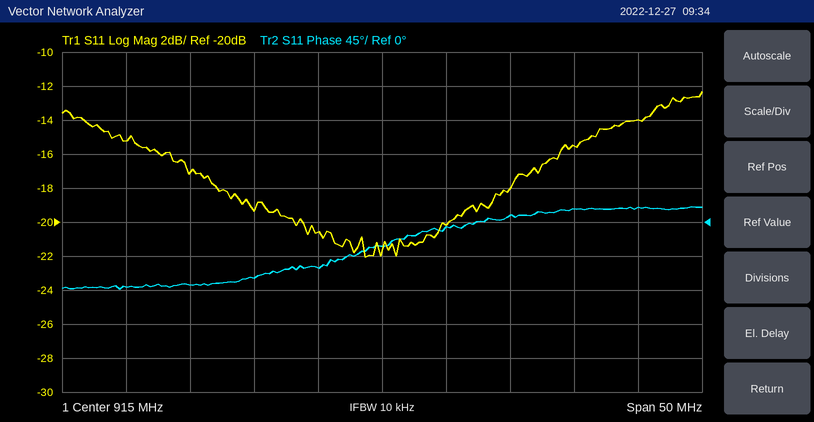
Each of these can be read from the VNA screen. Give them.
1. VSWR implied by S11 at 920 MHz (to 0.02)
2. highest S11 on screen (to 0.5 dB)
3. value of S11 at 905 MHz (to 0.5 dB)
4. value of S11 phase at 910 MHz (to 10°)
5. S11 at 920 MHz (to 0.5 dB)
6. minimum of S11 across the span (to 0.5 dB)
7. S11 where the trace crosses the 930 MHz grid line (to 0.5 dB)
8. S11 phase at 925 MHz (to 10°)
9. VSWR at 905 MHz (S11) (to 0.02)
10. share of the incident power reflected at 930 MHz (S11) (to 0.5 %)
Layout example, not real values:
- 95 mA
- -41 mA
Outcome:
- 1.22
- -12.5 dB
- -19.5 dB
- -60°
- -20.0 dB
- -22.0 dB
- -15.5 dB
- 10°
- 1.24
- 3.0 %
